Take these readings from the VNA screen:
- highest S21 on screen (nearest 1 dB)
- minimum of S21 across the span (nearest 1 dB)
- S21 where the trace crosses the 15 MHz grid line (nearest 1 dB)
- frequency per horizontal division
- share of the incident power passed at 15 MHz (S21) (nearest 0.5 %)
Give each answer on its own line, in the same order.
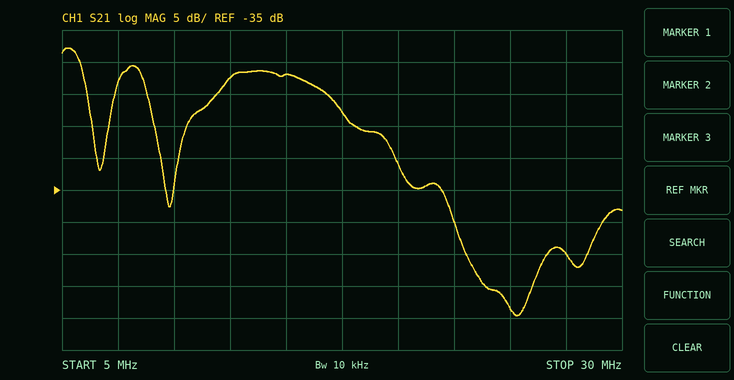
-13 dB
-55 dB
-17 dB
2.5 MHz
2.0 %
